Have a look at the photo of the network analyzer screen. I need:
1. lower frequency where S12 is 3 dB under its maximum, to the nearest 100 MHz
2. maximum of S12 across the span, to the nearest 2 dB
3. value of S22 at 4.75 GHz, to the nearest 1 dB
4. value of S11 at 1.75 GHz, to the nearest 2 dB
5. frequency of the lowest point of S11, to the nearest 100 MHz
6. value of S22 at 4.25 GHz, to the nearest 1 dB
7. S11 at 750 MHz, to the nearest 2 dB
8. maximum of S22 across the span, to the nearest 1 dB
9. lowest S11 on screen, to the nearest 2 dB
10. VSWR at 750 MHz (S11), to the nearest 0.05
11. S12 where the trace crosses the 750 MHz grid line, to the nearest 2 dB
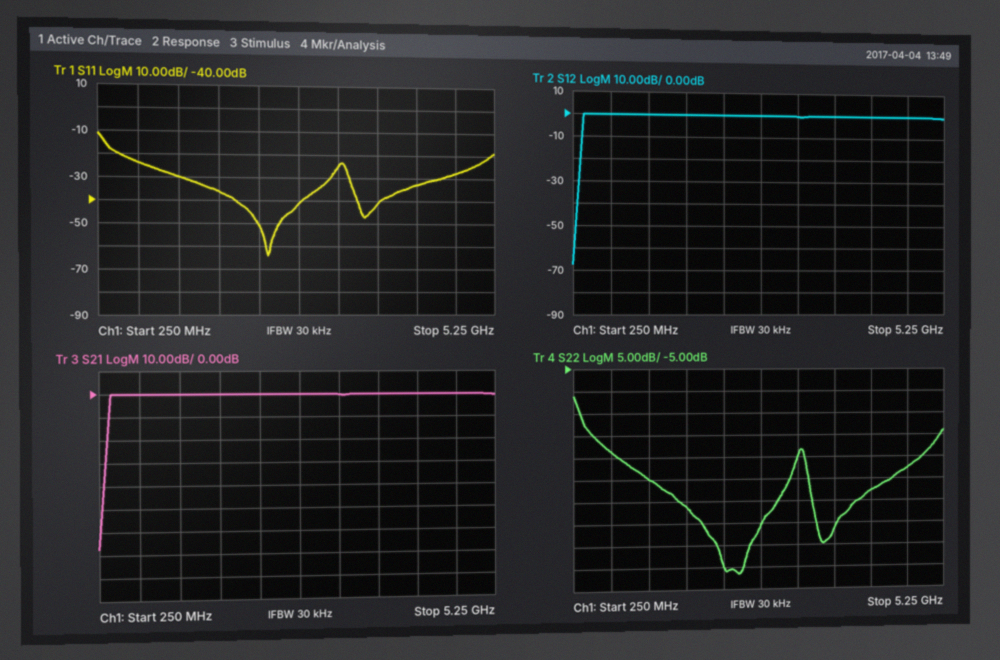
400 MHz
0 dB
-28 dB
-36 dB
2.4 GHz
-33 dB
-24 dB
-11 dB
-64 dB
1.15
0 dB
